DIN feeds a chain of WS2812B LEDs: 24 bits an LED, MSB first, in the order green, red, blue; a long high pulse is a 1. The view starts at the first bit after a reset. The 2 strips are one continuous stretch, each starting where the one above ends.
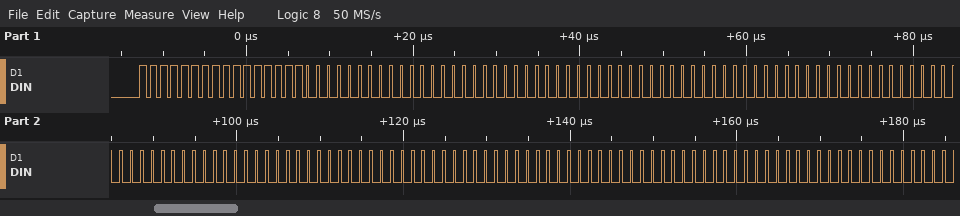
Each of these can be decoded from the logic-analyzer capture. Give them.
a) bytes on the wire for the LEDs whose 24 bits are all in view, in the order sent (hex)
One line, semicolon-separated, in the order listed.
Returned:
FF FF 00 00 00 00 00 00 00 00 00 00 00 00 00 00 00 00
